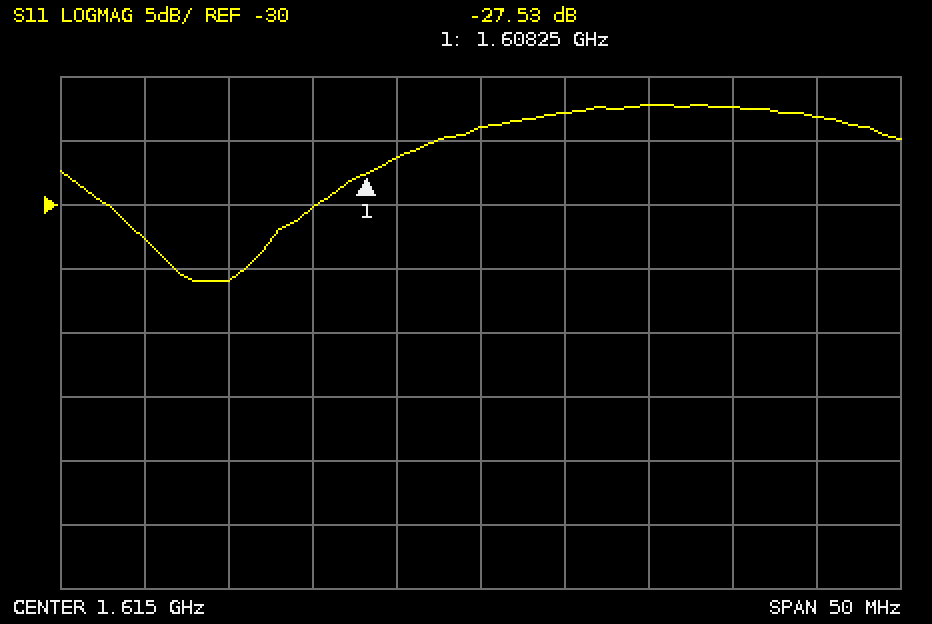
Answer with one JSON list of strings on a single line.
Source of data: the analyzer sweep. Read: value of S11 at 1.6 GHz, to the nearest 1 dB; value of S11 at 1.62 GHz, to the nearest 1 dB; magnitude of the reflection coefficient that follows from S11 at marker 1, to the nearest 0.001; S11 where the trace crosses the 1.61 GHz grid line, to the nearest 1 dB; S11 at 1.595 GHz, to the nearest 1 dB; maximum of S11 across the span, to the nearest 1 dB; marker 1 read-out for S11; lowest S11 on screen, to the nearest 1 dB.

["-36 dB", "-23 dB", "0.042", "-26 dB", "-33 dB", "-22 dB", "-27.53 dB", "-36 dB"]
